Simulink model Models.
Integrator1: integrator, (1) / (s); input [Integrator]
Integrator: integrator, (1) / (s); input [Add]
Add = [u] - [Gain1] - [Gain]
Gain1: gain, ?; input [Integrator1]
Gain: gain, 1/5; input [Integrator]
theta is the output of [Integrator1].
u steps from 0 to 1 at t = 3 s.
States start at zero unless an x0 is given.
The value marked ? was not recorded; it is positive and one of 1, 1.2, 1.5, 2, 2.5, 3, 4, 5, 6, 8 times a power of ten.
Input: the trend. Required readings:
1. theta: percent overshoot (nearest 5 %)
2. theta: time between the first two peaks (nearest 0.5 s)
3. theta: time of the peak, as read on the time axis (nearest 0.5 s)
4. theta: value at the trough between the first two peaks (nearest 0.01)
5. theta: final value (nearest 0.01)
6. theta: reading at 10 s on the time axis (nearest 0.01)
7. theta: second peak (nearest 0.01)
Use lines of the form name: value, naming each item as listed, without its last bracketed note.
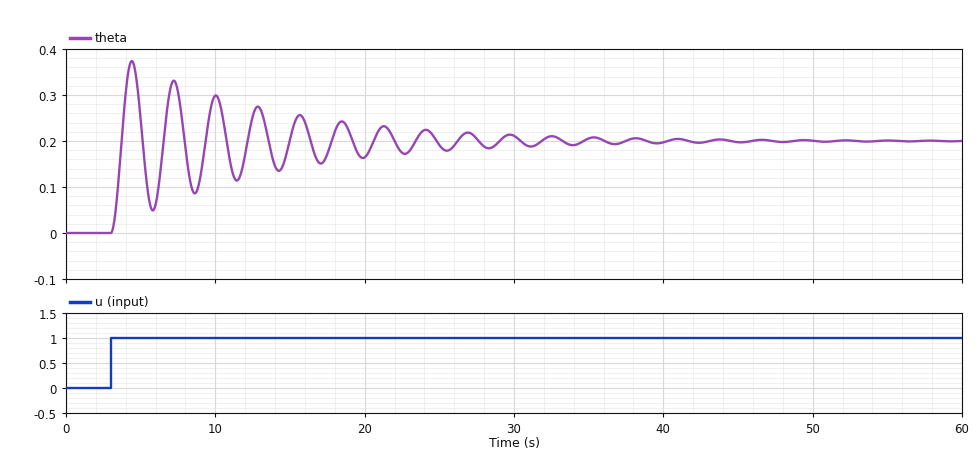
theta: percent overshoot: 85 %
theta: time between the first two peaks: 3.0 s
theta: time of the peak, as read on the time axis: 4.5 s
theta: value at the trough between the first two peaks: 0.05
theta: final value: 0.20
theta: reading at 10 s on the time axis: 0.30
theta: second peak: 0.33
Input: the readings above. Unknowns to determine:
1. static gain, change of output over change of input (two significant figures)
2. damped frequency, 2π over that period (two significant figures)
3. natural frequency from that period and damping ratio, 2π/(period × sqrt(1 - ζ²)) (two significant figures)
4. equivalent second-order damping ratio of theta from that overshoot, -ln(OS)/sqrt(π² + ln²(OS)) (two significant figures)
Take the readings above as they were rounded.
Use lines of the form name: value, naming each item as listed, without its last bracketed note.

static gain, change of output over change of input: 0.20
damped frequency, 2π over that period: 2.1 rad/s
natural frequency from that period and damping ratio, 2π/(period × sqrt(1 - ζ²)): 2.1 rad/s
equivalent second-order damping ratio of theta from that overshoot, -ln(OS)/sqrt(π² + ln²(OS)): 0.052
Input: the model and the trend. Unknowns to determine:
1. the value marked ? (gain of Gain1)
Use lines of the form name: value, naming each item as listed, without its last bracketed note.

the value marked ?: 5
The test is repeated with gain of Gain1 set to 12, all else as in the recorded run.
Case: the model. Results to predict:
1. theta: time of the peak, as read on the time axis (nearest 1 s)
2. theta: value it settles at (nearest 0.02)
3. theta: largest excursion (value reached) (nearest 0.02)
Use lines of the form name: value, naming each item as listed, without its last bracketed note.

theta: time of the peak, as read on the time axis: 4 s
theta: value it settles at: 0.08
theta: largest excursion (value reached): 0.16
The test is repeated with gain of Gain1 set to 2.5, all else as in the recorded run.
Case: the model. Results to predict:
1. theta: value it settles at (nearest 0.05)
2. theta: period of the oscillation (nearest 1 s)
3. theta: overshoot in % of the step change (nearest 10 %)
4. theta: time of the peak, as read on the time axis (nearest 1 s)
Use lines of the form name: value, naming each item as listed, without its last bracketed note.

theta: value it settles at: 0.40
theta: period of the oscillation: 4 s
theta: overshoot in % of the step change: 80 %
theta: time of the peak, as read on the time axis: 5 s
